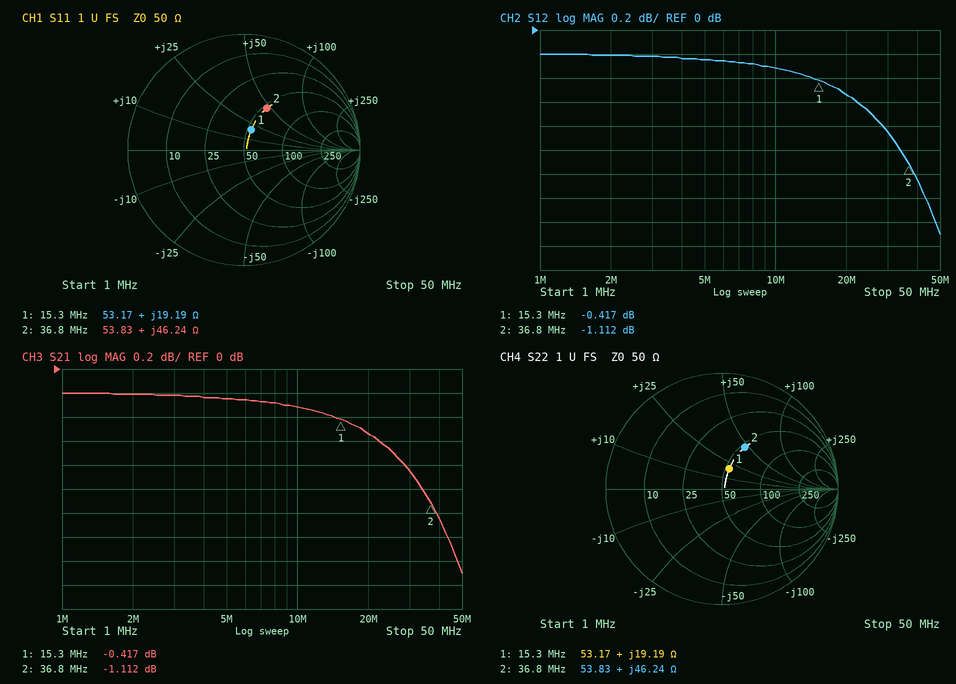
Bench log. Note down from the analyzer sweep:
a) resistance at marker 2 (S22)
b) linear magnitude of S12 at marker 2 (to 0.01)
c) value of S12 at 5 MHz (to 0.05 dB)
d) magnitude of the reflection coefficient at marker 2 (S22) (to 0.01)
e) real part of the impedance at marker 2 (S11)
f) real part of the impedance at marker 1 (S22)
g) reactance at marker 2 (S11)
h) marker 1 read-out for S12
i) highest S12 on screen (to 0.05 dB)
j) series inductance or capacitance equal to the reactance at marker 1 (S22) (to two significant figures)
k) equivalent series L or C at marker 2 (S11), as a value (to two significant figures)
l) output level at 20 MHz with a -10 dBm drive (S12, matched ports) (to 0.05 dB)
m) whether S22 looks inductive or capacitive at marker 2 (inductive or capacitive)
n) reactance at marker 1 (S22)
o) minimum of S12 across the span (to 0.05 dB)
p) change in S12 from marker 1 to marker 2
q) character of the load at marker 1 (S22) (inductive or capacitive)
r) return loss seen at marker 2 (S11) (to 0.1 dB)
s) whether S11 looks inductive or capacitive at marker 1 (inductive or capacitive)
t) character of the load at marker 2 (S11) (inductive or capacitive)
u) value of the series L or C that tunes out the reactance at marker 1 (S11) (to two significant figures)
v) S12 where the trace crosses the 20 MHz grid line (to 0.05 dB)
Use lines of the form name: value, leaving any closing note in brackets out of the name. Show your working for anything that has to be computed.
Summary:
resistance at marker 2: 53.83 Ω
linear magnitude of S12 at marker 2: 10^(-1.112/20) ≈ 0.88
value of S12 at 5 MHz: -0.25 dB
magnitude of the reflection coefficient at marker 2 (S22): 0.41
real part of the impedance at marker 2: 53.83 Ω
real part of the impedance at marker 1: 53.17 Ω
reactance at marker 2: +46.24 Ω
marker 1 read-out for S12: -0.417 dB
highest S12 on screen: -0.20 dB
series inductance or capacitance equal to the reactance at marker 1 (S22): L = 19.19 Ω/(2π × 15.3 MHz) ≈ 200 nH
equivalent series L or C at marker 2 (S11), as a value: L = 46.24 Ω/(2π × 36.8 MHz) ≈ 200 nH
output level at 20 MHz with a -10 dBm drive (S12, matched ports): -10 dBm + (-0.55 dB) = -10.55 dBm
whether S22 looks inductive or capacitive at marker 2: inductive
reactance at marker 1: +19.19 Ω
minimum of S12 across the span: -1.70 dB
change in S12 from marker 1 to marker 2: -1.112 − (-0.417) = -0.695 dB
character of the load at marker 1 (S22): inductive
return loss seen at marker 2 (S11): 7.8 dB
whether S11 looks inductive or capacitive at marker 1: inductive
character of the load at marker 2 (S11): inductive
value of the series L or C that tunes out the reactance at marker 1 (S11): C = 1/(2π × 15.3 MHz × 19.19 Ω) ≈ 542 pF, so 540 pF to two significant figures
S12 where the trace crosses the 20 MHz grid line: -0.55 dB
